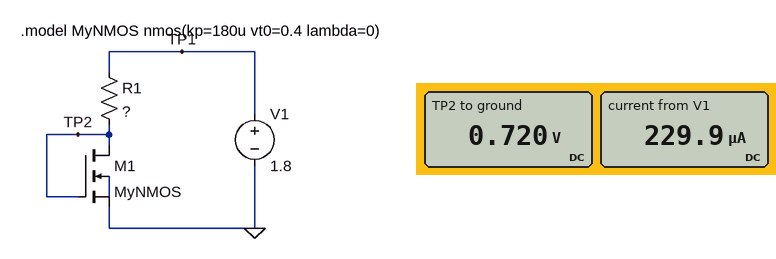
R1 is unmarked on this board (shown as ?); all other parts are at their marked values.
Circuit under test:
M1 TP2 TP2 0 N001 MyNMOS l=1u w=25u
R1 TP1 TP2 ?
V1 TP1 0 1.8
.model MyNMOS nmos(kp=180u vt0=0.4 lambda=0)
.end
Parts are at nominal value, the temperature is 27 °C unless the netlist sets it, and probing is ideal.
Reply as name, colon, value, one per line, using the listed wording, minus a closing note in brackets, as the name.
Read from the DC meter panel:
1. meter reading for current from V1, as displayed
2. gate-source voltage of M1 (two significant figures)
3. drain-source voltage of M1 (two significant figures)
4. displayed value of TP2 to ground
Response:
meter reading for current from V1, as displayed: 229.9 µA
gate-source voltage of M1: 720 mV
drain-source voltage of M1: 720 mV
displayed value of TP2 to ground: 0.720 V
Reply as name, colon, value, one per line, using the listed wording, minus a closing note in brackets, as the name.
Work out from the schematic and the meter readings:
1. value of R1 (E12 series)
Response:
value of R1: 4.7 kΩ
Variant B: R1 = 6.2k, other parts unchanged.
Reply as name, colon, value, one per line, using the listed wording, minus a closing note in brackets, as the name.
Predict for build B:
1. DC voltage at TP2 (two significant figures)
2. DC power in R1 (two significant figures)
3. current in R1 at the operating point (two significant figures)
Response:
DC voltage at TP2: 680 mV
DC power in R1: 200 µW
current in R1 at the operating point: 180 µA
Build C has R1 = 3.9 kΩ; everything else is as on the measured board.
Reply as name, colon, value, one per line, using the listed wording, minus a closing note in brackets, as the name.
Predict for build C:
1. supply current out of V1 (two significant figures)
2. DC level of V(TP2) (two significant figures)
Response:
supply current out of V1: 270 µA
DC level of V(TP2): 750 mV
